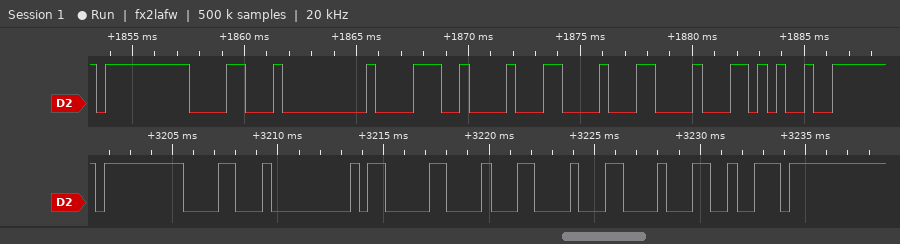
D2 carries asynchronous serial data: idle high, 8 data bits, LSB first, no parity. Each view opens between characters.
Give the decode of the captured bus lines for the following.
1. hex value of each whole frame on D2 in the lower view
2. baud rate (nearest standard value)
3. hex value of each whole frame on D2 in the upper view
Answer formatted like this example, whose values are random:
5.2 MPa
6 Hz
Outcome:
FF, 18, 00, 83, 88, 88, 88, 72
2400 baud
FF, 18, 00, 38, 88, 88, 88, 25
